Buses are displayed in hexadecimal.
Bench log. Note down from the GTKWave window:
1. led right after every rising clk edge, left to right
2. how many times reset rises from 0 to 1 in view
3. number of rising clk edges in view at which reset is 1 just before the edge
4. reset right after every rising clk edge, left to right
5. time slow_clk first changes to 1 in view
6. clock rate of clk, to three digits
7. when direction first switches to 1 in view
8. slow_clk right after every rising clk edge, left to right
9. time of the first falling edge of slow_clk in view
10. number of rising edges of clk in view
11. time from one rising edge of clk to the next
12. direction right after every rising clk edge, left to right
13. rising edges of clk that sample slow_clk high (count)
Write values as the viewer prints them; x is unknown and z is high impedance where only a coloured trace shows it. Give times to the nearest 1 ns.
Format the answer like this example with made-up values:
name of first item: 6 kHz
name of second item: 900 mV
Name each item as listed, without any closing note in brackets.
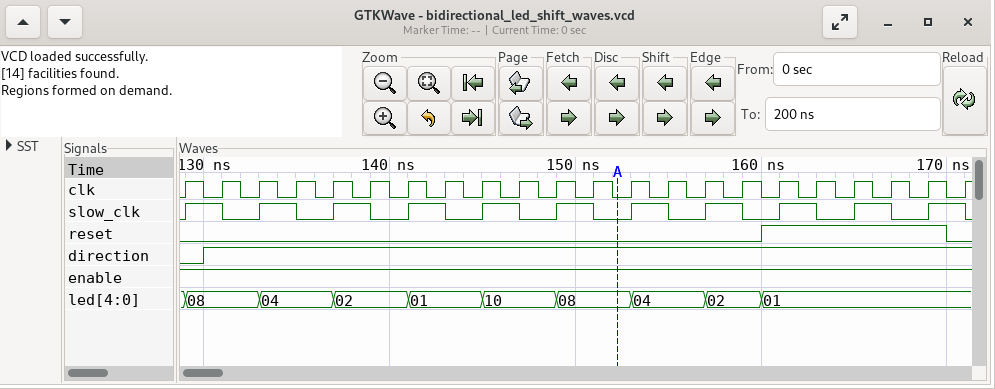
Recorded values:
led right after every rising clk edge, left to right: 08, 08, 04, 04, 02, 02, 01, 01, 10, 10, 08, 08, 04, 04, 02, 02, 01, 01, 01, 01, 01, 01
how many times reset rises from 0 to 1 in view: 1
number of rising clk edges in view at which reset is 1 just before the edge: 5
reset right after every rising clk edge, left to right: 0 0 0 0 0 0 0 0 0 0 0 0 0 0 0 0 1 1 1 1 1 0
time slow_clk first changes to 1 in view: 129 ns
clock rate of clk, to three digits: 500 MHz
when direction first switches to 1 in view: 130 ns
slow_clk right after every rising clk edge, left to right: 1 0 1 0 1 0 1 0 1 0 1 0 1 0 1 0 1 0 1 0 1 0
time of the first falling edge of slow_clk in view: 131 ns
number of rising edges of clk in view: 22
time from one rising edge of clk to the next: 2 ns
direction right after every rising clk edge, left to right: 0 1 1 1 1 1 1 1 1 1 1 1 1 1 1 1 1 1 1 1 1 1
rising edges of clk that sample slow_clk high: 11
